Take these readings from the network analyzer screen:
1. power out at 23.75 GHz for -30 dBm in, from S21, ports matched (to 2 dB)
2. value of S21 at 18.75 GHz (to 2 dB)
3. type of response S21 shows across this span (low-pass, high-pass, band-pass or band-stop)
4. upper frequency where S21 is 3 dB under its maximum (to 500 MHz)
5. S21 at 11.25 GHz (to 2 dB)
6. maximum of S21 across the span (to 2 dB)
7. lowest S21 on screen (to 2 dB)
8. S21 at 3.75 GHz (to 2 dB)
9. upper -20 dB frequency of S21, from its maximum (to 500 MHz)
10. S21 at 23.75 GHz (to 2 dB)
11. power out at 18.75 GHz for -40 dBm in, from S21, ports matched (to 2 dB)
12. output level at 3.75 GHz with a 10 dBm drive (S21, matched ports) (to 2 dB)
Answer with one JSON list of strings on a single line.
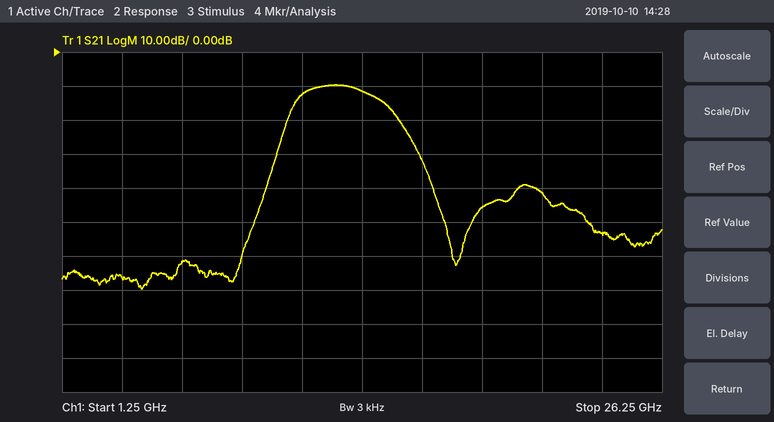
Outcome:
["-84 dBm", "-46 dB", "band-pass", "14.0 GHz", "-12 dB", "-10 dB", "-70 dB", "-66 dB", "16.0 GHz", "-54 dB", "-86 dBm", "-56 dBm"]
